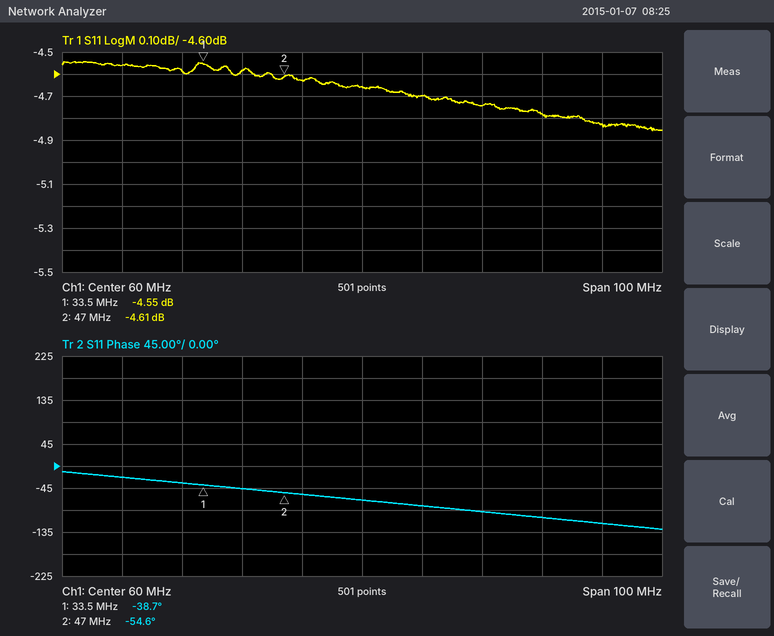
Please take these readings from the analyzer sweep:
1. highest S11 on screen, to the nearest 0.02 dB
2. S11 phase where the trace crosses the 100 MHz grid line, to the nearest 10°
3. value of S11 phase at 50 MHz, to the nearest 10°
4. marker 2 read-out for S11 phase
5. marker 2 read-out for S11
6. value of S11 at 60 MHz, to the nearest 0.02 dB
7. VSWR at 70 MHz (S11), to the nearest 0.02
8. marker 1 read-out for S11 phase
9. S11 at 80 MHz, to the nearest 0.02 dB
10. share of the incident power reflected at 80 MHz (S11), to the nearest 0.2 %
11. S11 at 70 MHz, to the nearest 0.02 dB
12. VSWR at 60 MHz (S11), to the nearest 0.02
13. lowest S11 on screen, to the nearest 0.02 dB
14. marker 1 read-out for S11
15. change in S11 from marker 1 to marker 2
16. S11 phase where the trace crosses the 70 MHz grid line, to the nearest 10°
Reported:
-4.54 dB
-120°
-60°
-54.6°
-4.61 dB
-4.66 dB
3.78
-38.7°
-4.74 dB
33.6 %
-4.70 dB
3.82
-4.86 dB
-4.55 dB
-0.06 dB
-80°
